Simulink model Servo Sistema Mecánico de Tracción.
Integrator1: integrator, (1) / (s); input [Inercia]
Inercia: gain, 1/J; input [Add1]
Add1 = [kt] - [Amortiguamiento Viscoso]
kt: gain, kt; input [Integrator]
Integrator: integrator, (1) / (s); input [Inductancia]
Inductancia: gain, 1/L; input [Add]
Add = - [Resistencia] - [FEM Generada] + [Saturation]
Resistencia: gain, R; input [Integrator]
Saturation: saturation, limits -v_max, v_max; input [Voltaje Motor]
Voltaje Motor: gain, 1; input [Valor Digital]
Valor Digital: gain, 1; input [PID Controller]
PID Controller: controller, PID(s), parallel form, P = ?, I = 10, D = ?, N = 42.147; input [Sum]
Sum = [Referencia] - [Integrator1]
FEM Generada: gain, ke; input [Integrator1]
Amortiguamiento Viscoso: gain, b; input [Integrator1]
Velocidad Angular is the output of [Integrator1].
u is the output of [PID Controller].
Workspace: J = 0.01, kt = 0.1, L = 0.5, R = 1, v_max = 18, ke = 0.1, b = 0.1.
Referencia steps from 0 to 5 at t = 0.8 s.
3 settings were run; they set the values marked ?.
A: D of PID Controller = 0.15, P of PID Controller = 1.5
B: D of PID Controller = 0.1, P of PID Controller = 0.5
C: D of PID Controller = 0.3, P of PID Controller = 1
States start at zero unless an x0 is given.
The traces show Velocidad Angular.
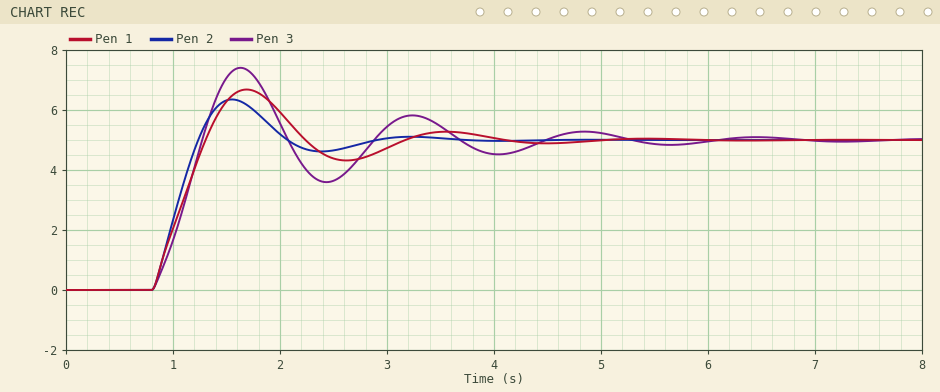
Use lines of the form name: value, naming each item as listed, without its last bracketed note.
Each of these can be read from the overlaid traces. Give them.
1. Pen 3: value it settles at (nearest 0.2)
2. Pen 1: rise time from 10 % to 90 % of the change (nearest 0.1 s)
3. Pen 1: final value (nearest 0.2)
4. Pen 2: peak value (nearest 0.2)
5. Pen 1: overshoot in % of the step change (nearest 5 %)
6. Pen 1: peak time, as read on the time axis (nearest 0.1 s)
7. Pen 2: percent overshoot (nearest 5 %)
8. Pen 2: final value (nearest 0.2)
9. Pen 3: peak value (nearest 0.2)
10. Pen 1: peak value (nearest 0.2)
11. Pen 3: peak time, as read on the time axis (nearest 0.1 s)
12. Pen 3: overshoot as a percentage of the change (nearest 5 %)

Pen 3: value it settles at: 5.0
Pen 1: rise time from 10 % to 90 % of the change: 0.4 s
Pen 1: final value: 5.0
Pen 2: peak value: 6.4
Pen 1: overshoot in % of the step change: 35 %
Pen 1: peak time, as read on the time axis: 1.7 s
Pen 2: percent overshoot: 25 %
Pen 2: final value: 5.0
Pen 3: peak value: 7.4
Pen 1: peak value: 6.6
Pen 3: peak time, as read on the time axis: 1.6 s
Pen 3: overshoot as a percentage of the change: 50 %
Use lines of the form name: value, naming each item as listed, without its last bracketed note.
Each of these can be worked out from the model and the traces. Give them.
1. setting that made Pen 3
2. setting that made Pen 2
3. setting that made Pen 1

setting that made Pen 3: B
setting that made Pen 2: A
setting that made Pen 1: C
